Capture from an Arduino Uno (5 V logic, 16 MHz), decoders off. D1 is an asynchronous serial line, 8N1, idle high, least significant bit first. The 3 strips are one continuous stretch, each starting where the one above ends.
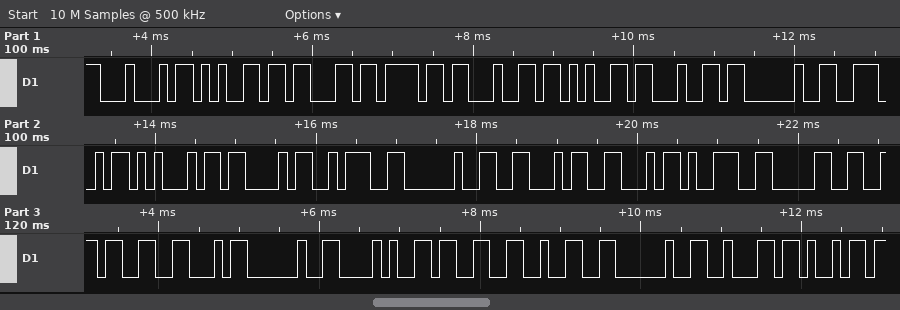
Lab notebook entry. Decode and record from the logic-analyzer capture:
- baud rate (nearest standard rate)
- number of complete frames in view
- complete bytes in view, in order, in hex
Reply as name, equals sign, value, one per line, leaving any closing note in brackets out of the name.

baud rate = 9600 baud
number of complete frames in view = 26
complete bytes in view, in order, in hex = 0x44 0x65 0x63 0x6F 0x64 0x65 0x64 0x20 0x4E 0x45 0x43 0x3A 0x20 0x46 0x46 0x39 0x30 0x36 0x46 0x20 0x28 0x33 0x32 0x20 0x62 0x69
